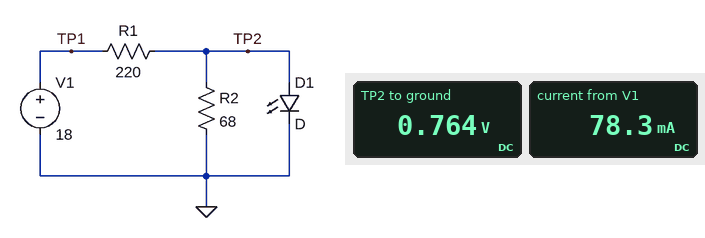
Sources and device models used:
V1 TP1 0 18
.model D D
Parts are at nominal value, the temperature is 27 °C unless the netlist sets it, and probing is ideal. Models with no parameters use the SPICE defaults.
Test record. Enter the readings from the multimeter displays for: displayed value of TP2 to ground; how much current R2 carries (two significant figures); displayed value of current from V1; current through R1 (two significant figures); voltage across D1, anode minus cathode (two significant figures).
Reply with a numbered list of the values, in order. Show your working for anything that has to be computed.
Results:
1. 0.764 V
2. (764 mV) / 68 Ω = 11 mA
3. 78.3 mA
4. (18 V - 764 mV) / 220 Ω = 78 mA
5. 764 mV = 760 mV
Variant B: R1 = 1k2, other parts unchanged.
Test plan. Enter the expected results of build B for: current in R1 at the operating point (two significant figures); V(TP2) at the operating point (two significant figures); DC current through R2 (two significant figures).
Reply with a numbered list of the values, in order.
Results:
1. 14 mA
2. 690 mV
3. 10 mA
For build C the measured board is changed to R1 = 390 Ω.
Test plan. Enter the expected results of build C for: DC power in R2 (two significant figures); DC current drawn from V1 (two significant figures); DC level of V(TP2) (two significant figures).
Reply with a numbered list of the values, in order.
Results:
1. 8.2 mW
2. 44 mA
3. 750 mV
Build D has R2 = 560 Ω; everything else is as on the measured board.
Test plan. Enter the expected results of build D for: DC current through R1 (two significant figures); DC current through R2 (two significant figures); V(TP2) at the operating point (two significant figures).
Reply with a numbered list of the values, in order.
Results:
1. 78 mA
2. 1.4 mA
3. 770 mV
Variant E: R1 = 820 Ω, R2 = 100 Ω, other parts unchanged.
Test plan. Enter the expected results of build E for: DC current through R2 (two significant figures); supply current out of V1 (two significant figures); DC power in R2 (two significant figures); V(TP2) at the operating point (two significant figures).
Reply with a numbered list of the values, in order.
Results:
1. 7.2 mA
2. 21 mA
3. 5.2 mW
4. 720 mV
